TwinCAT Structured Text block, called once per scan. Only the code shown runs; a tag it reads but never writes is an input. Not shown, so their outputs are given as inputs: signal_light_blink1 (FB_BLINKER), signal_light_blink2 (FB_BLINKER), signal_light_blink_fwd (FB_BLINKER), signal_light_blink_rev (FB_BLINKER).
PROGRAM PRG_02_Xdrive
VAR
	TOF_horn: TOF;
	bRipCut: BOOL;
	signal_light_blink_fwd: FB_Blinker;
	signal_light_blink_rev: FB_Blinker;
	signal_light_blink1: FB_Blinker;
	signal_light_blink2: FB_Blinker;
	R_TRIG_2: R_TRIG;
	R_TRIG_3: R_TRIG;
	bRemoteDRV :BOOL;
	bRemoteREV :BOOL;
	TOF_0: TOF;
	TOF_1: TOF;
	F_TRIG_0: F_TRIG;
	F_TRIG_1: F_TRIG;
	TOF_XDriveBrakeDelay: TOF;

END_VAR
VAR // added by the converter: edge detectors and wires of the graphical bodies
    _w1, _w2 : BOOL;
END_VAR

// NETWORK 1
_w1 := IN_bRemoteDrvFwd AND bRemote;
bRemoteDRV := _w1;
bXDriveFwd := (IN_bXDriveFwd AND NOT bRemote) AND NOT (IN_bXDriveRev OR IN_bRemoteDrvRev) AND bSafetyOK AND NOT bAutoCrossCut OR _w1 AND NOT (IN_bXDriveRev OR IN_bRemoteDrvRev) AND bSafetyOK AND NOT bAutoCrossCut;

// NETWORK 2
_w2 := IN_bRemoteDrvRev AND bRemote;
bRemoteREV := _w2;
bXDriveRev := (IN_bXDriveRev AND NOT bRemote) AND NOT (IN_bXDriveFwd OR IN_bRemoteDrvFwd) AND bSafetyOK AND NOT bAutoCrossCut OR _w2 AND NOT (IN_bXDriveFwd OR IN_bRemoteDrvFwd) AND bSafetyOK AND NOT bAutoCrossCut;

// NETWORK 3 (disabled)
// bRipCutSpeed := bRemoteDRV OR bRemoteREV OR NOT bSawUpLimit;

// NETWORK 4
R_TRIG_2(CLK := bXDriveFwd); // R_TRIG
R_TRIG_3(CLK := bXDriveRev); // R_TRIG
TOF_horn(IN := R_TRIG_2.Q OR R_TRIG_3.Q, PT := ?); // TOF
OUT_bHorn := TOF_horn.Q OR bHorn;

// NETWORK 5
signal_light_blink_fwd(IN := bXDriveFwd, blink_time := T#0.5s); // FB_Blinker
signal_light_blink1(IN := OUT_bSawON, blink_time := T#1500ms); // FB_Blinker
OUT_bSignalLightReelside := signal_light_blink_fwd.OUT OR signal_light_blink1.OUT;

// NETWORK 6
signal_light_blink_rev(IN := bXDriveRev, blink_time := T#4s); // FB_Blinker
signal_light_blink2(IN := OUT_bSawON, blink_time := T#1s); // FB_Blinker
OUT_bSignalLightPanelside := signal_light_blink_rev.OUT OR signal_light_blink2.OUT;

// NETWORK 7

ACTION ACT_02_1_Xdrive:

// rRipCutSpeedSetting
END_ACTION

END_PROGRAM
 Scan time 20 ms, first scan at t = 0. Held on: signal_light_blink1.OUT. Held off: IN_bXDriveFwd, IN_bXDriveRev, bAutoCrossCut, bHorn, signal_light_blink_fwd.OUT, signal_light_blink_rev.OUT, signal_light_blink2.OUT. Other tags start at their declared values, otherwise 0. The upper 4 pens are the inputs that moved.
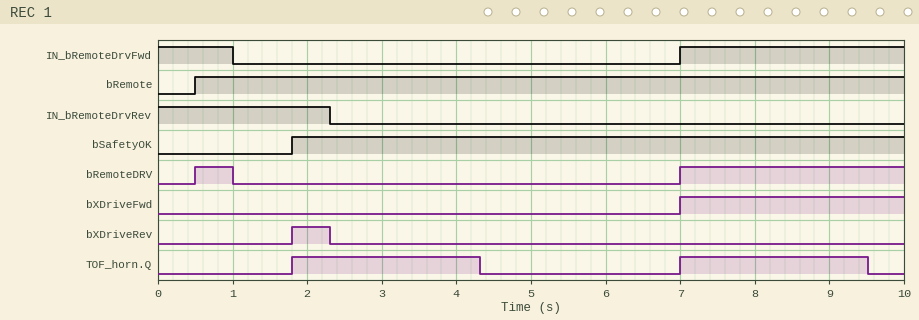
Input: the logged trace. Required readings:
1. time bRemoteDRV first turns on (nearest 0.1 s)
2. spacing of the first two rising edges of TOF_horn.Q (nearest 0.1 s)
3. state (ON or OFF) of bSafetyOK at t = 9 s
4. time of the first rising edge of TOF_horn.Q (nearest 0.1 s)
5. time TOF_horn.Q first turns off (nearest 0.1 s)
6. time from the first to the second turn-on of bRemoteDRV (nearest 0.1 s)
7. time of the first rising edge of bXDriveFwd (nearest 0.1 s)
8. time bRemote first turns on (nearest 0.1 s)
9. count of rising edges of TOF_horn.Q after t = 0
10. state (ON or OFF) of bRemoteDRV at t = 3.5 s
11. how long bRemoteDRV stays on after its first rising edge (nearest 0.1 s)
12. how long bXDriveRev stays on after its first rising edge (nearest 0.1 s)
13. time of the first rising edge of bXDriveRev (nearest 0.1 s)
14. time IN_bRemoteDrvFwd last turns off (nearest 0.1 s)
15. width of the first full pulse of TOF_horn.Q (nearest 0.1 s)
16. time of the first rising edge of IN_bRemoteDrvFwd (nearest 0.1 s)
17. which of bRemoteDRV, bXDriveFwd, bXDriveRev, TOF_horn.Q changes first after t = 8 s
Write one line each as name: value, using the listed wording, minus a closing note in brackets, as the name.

time bRemoteDRV first turns on: 0.5 s
spacing of the first two rising edges of TOF_horn.Q: 5.2 s
state (ON or OFF) of bSafetyOK at t = 9 s: ON
time of the first rising edge of TOF_horn.Q: 1.8 s
time TOF_horn.Q first turns off: 4.3 s
time from the first to the second turn-on of bRemoteDRV: 6.5 s
time of the first rising edge of bXDriveFwd: 7.0 s
time bRemote first turns on: 0.5 s
count of rising edges of TOF_horn.Q after t = 0: 2
state (ON or OFF) of bRemoteDRV at t = 3.5 s: OFF
how long bRemoteDRV stays on after its first rising edge: 0.5 s
how long bXDriveRev stays on after its first rising edge: 0.5 s
time of the first rising edge of bXDriveRev: 1.8 s
time IN_bRemoteDrvFwd last turns off: 1.0 s
width of the first full pulse of TOF_horn.Q: 2.5 s
time of the first rising edge of IN_bRemoteDrvFwd: 7.0 s
which of bRemoteDRV, bXDriveFwd, bXDriveRev, TOF_horn.Q changes first after t = 8 s: TOF_horn.Q
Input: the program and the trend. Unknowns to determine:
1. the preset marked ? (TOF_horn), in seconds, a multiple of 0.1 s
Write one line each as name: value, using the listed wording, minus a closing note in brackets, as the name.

the preset marked ? (TOF_horn), in seconds, a multiple of 0.1 s: 2.5 s
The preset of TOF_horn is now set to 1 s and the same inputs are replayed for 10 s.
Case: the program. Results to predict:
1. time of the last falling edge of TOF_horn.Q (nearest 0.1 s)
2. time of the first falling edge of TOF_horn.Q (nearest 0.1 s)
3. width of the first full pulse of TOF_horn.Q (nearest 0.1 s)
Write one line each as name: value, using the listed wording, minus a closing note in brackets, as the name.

time of the last falling edge of TOF_horn.Q: 8.0 s
time of the first falling edge of TOF_horn.Q: 2.8 s
width of the first full pulse of TOF_horn.Q: 1.0 s
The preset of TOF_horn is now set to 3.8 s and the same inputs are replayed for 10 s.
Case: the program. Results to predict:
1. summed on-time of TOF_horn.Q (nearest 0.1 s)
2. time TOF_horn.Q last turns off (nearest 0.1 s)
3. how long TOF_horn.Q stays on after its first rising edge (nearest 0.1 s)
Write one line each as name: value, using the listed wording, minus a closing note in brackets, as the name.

summed on-time of TOF_horn.Q: 6.8 s
time TOF_horn.Q last turns off: 5.6 s
how long TOF_horn.Q stays on after its first rising edge: 3.8 s
